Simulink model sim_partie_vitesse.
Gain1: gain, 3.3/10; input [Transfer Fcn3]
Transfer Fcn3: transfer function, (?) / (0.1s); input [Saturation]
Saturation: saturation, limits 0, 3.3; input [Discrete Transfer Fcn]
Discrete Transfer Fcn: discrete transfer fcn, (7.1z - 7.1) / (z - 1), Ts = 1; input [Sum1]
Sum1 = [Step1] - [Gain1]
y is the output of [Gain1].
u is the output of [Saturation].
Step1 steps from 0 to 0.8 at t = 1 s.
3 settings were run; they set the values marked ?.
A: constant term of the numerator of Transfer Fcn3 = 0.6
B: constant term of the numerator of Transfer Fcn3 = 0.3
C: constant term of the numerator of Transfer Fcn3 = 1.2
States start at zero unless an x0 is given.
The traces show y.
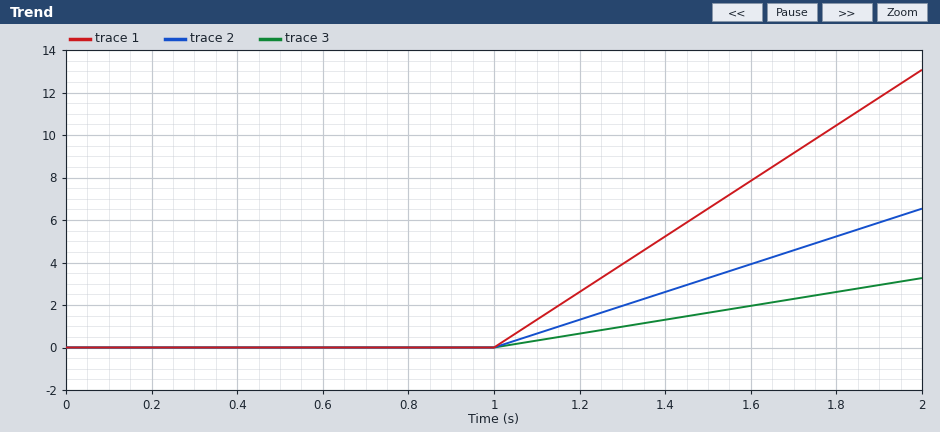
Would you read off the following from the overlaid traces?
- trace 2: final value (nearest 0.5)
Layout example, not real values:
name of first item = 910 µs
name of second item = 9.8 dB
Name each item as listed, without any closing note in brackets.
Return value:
trace 2: final value = 6.5
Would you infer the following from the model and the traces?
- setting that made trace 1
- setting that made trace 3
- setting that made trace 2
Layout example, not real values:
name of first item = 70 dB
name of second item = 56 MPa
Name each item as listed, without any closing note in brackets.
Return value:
setting that made trace 1 = C
setting that made trace 3 = B
setting that made trace 2 = A
